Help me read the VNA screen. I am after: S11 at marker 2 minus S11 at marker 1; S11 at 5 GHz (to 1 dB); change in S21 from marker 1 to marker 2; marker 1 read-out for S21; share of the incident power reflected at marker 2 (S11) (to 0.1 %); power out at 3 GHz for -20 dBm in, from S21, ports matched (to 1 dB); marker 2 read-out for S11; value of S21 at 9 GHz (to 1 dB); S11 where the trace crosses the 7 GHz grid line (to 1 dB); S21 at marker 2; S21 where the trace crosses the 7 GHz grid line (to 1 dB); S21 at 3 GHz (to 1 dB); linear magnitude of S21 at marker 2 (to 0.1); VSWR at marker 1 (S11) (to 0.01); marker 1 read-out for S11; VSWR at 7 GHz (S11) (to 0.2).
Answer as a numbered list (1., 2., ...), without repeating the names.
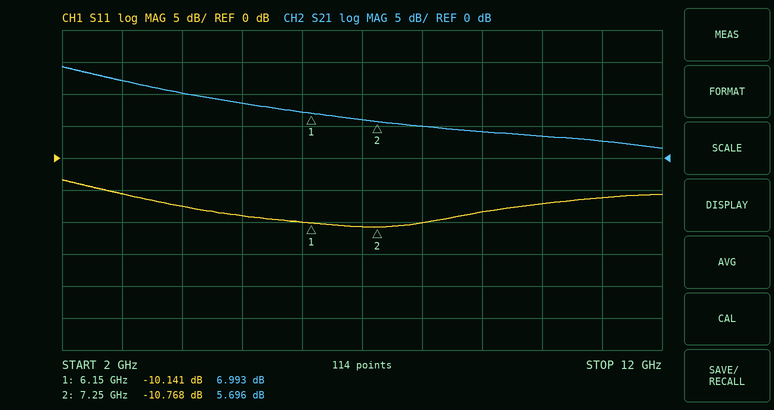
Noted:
1. -0.627 dB
2. -9 dB
3. -1.297 dB
4. 6.993 dB
5. 8.4 %
6. -8 dBm
7. -10.768 dB
8. 4 dB
9. -11 dB
10. 5.696 dB
11. 6 dB
12. 12 dB
13. 1.9
14. 1.90
15. -10.141 dB
16. 1.8
